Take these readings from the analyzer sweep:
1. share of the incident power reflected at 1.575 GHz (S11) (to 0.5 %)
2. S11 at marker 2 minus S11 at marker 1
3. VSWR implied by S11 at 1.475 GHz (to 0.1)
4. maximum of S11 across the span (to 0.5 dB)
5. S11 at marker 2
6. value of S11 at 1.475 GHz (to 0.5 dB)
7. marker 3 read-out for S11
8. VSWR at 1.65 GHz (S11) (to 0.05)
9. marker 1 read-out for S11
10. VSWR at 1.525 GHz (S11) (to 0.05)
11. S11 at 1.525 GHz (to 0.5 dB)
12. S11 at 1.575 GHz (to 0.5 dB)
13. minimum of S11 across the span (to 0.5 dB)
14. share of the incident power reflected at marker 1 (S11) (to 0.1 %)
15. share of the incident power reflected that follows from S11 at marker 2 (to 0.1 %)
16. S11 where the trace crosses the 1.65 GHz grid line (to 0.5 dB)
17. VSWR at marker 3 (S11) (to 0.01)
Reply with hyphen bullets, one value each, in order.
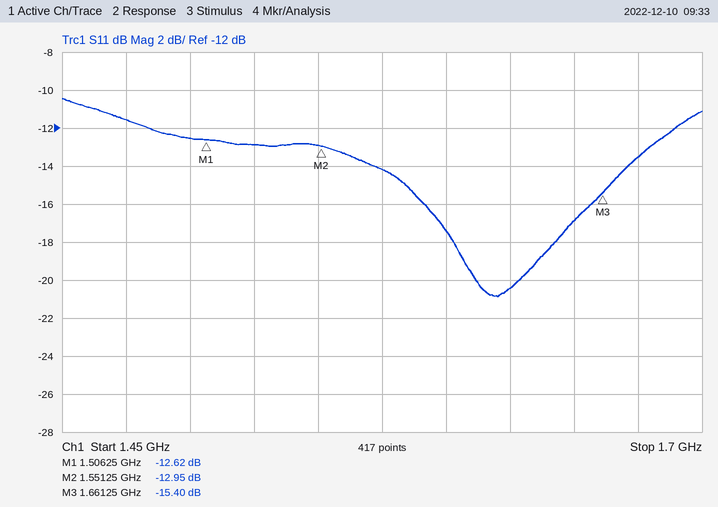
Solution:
- 4.0 %
- -0.33 dB
- 1.7
- -10.5 dB
- -12.95 dB
- -11.5 dB
- -15.40 dB
- 1.35
- -12.62 dB
- 1.60
- -13.0 dB
- -14.0 dB
- -21.0 dB
- 5.5 %
- 5.1 %
- -17.0 dB
- 1.41
